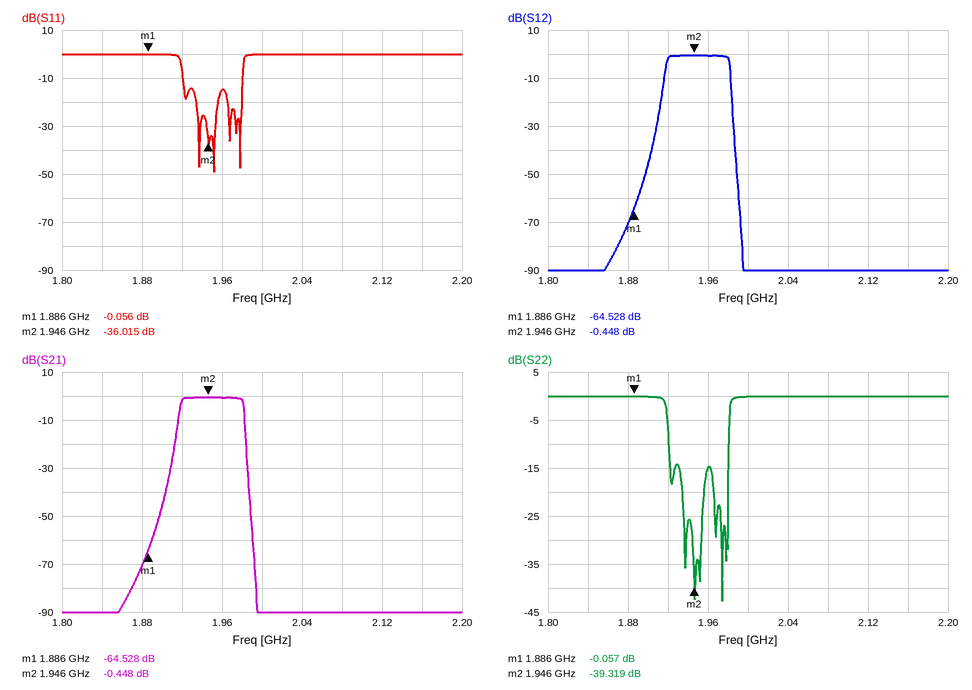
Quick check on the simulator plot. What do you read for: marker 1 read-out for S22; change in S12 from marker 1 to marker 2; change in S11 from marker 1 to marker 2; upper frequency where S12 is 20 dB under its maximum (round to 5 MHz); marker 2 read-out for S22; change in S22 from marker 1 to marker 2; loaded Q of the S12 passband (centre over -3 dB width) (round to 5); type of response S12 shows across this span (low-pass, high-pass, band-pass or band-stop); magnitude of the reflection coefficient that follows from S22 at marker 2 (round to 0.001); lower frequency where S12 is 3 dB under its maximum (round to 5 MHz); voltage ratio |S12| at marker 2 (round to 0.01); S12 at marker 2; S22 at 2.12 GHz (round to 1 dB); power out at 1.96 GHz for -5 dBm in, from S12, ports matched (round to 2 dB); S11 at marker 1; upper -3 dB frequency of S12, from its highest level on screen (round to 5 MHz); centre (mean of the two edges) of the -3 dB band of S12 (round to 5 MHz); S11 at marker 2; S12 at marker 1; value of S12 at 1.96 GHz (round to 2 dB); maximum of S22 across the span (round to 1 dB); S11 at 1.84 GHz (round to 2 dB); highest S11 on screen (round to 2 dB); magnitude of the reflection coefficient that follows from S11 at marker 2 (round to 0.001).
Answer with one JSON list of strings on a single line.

["-0.057 dB", "64.080 dB", "-35.959 dB", "1.985 GHz", "-39.319 dB", "-39.262 dB", "30", "band-pass", "0.011", "1.920 GHz", "0.95", "-0.448 dB", "0 dB", "-6 dBm", "-0.056 dB", "1.980 GHz", "1.950 GHz", "-36.015 dB", "-64.528 dB", "0 dB", "0 dB", "0 dB", "0 dB", "0.016"]
